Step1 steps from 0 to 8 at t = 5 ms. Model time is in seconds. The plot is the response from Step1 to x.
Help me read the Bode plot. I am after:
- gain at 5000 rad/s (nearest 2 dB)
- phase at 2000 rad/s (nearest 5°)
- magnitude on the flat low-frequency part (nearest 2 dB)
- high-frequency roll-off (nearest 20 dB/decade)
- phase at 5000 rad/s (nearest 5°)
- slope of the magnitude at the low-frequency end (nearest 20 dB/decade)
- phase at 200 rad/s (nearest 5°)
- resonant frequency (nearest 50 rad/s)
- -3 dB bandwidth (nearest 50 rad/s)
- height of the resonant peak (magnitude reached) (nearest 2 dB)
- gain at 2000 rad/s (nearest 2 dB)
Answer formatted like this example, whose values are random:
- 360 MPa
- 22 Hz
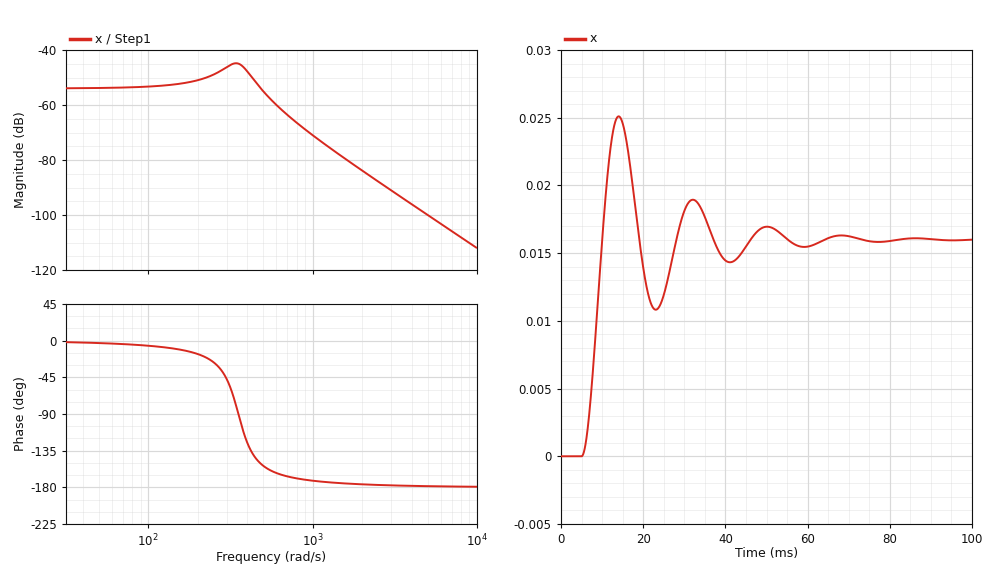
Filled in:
- -100 dB
- -175°
- -54 dB
- -40 dB/decade
- -180°
- 0 dB/decade
- -15°
- 350 rad/s
- 550 rad/s
- -44 dB
- -84 dB
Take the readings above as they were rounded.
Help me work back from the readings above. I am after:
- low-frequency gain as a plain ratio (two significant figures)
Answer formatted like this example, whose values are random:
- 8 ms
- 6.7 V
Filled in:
- 0.0020
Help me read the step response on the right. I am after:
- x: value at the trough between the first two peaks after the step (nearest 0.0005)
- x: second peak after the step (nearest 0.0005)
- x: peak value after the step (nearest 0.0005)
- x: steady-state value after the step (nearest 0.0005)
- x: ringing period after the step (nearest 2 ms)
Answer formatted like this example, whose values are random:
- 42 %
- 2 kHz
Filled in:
- 0.0110
- 0.0190
- 0.0250
- 0.0160
- 18 ms
